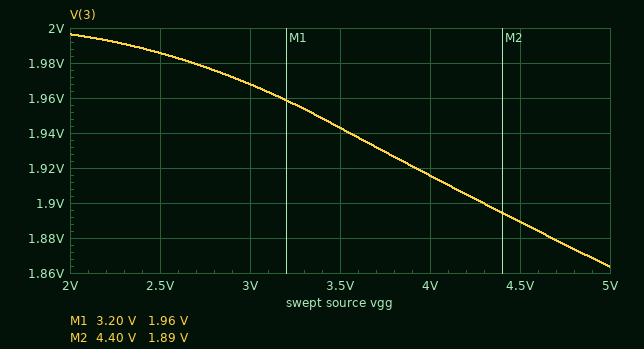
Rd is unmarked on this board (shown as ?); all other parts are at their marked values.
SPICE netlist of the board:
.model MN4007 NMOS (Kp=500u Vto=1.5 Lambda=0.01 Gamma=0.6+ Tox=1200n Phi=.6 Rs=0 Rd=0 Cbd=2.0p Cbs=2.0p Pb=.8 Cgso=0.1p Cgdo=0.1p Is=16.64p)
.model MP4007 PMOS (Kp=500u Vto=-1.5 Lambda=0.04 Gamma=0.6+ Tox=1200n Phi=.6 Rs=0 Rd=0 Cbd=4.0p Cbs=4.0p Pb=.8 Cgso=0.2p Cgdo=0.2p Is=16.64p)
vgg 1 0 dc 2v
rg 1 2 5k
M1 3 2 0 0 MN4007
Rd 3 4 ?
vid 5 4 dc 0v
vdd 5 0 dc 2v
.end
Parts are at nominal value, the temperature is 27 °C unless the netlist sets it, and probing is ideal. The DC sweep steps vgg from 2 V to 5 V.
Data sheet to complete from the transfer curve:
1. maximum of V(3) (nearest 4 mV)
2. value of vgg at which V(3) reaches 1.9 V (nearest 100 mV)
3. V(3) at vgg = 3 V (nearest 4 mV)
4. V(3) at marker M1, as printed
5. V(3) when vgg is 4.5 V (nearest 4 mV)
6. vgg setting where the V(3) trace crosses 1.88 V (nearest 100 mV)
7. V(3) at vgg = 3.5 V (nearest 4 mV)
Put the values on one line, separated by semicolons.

1.996 V; 4.3 V; 1.968 V; 1.96 V; 1.888 V; 4.7 V; 1.944 V
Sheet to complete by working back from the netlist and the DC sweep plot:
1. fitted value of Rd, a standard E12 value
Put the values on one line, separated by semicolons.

56 Ω
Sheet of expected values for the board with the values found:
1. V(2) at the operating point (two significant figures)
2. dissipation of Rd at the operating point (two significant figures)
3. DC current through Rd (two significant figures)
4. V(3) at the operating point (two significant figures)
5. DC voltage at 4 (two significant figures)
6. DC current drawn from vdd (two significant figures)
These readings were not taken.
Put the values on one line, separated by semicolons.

2.0 V; 230 nW; 64 µA; 2.0 V; 2.0 V; 64 µA
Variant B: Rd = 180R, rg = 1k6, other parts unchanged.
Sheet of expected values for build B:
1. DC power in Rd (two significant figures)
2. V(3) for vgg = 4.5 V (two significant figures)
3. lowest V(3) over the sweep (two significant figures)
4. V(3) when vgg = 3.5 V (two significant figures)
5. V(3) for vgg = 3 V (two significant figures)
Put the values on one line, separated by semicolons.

730 nW; 1.7 V; 1.6 V; 1.8 V; 1.9 V
